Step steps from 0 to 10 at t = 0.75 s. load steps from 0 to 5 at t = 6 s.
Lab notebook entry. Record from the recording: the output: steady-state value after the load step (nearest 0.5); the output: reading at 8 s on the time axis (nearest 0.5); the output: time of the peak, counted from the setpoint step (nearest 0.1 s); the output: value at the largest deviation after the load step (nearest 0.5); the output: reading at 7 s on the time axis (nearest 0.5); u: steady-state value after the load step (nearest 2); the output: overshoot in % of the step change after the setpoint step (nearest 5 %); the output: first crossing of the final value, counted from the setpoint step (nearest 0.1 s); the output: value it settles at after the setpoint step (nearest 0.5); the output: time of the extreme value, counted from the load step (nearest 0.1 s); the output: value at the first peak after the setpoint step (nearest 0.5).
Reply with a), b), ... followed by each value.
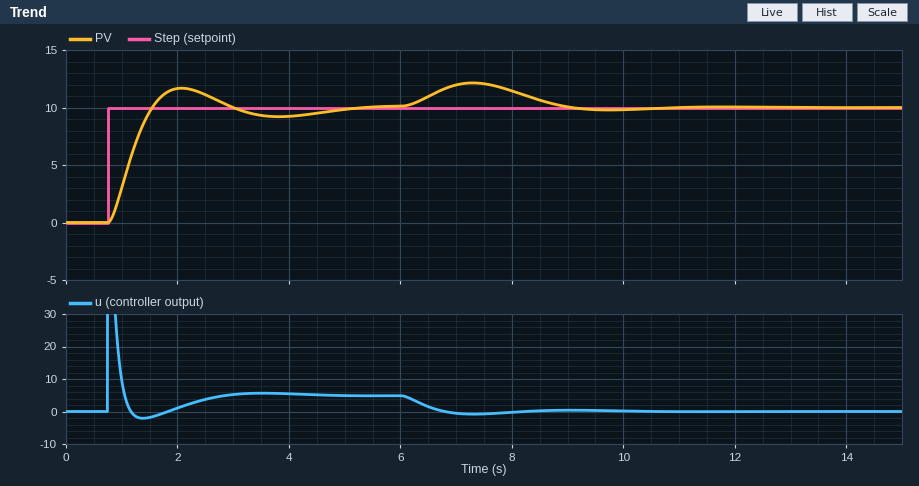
a) 10.0
b) 11.5
c) 1.3 s
d) 12.0
e) 12.0
f) 0
g) 15 %
h) 0.8 s
i) 10.0
j) 1.3 s
k) 11.5
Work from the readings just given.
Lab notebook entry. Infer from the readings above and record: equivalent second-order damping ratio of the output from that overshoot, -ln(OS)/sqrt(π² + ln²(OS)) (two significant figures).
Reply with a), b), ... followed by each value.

a) 0.52
